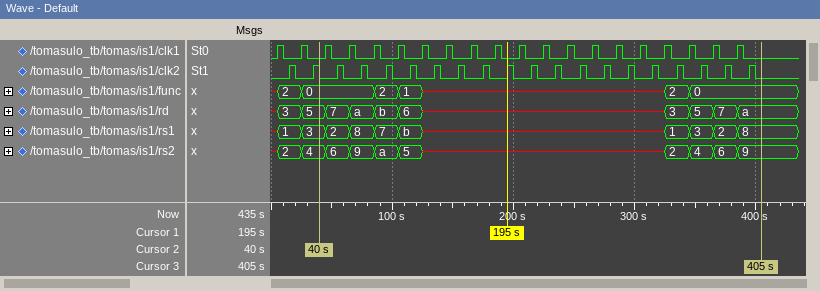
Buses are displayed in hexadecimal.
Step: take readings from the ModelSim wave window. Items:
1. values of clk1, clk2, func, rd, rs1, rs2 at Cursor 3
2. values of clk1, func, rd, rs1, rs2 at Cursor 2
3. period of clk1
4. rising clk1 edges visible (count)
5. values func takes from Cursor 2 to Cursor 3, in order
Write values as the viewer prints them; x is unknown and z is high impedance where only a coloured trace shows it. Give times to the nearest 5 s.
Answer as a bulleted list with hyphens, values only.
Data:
- clk1=0, clk2=0, func=0, rd=a, rs1=8, rs2=9
- clk1=0, func=0, rd=5, rs1=3, rs2=4
- 20 s
- 20
- 0, 2, 1, x, 2, 0
